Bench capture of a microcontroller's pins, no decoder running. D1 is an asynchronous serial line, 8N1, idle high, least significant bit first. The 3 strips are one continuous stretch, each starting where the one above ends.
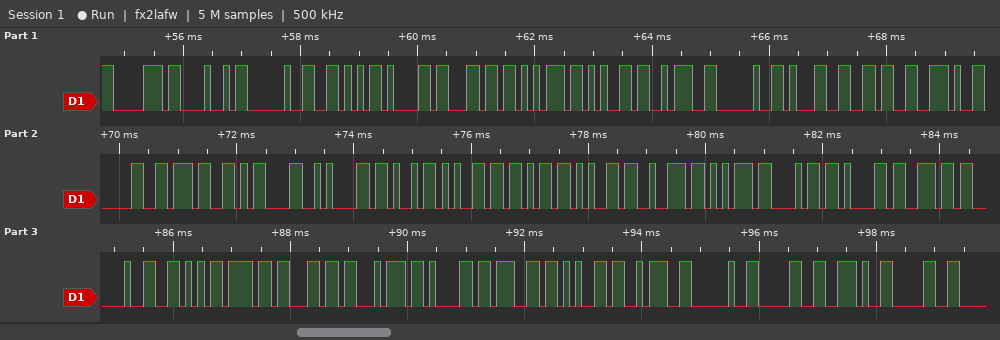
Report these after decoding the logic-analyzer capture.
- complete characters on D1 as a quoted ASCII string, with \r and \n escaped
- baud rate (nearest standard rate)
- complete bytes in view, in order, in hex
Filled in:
"pH Value: 16.07\r\nKekeruhan Voltage: 0.0"
9600 baud
70 48 20 56 61 6C 75 65 3A 20 31 36 2E 30 37 0D 0A 4B 65 6B 65 72 75 68 61 6E 20 56 6F 6C 74 61 67 65 3A 20 30 2E 30
